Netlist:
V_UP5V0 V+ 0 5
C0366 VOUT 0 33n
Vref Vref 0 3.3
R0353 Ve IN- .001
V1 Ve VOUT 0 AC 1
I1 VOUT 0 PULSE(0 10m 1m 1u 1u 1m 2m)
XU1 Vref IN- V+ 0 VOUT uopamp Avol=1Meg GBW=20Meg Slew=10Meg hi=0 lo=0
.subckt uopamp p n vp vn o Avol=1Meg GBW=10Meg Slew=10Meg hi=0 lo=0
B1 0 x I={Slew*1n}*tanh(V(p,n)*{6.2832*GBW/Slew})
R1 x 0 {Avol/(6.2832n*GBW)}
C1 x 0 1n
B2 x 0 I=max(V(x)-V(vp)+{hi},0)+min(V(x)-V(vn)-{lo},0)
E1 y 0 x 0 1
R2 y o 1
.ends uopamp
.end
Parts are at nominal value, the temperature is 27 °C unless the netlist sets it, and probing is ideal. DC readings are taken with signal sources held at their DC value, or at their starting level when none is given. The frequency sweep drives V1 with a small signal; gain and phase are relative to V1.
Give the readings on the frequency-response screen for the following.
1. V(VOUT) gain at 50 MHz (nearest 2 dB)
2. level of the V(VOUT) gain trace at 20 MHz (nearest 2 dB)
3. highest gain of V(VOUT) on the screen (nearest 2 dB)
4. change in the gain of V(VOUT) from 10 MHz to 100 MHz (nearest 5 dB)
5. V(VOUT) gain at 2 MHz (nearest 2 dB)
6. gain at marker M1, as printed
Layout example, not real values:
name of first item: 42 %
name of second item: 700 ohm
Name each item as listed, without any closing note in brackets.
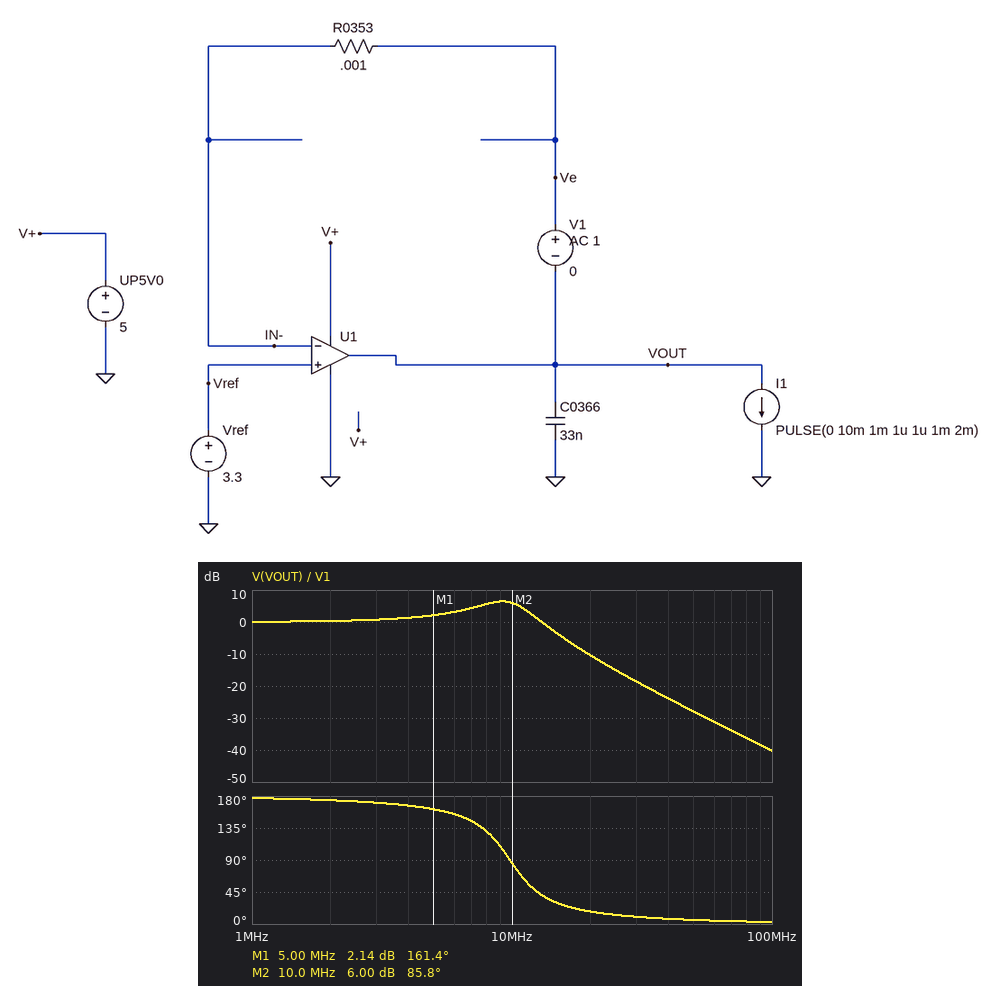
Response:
V(VOUT) gain at 50 MHz: -28 dB
level of the V(VOUT) gain trace at 20 MHz: -10 dB
highest gain of V(VOUT) on the screen: 6 dB
change in the gain of V(VOUT) from 10 MHz to 100 MHz: -45 dB
V(VOUT) gain at 2 MHz: 0 dB
gain at marker M1, as printed: 2.14 dB
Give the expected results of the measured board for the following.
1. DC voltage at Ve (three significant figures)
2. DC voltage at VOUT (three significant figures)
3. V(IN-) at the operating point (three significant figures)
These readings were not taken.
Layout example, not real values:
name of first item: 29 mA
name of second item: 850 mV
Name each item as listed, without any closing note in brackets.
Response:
DC voltage at Ve: 3.30 V
DC voltage at VOUT: 3.30 V
V(IN-) at the operating point: 3.30 V
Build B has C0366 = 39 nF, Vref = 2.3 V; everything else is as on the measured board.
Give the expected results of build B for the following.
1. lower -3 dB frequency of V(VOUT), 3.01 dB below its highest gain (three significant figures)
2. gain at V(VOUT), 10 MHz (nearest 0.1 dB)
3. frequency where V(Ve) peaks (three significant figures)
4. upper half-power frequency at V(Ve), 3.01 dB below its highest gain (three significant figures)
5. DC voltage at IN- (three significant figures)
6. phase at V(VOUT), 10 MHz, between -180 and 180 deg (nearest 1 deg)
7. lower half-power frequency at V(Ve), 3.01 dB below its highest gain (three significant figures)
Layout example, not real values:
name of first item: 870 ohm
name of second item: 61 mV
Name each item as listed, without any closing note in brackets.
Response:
lower -3 dB frequency of V(VOUT), 3.01 dB below its highest gain: 6.11 MHz
gain at V(VOUT), 10 MHz: 5.2 dB
frequency where V(Ve) peaks: 9.45 MHz
upper half-power frequency at V(Ve), 3.01 dB below its highest gain: 12.9 MHz
DC voltage at IN-: 2.30 V
phase at V(VOUT), 10 MHz, between -180 and 180 deg: 66 deg
lower half-power frequency at V(Ve), 3.01 dB below its highest gain: 7.71 MHz
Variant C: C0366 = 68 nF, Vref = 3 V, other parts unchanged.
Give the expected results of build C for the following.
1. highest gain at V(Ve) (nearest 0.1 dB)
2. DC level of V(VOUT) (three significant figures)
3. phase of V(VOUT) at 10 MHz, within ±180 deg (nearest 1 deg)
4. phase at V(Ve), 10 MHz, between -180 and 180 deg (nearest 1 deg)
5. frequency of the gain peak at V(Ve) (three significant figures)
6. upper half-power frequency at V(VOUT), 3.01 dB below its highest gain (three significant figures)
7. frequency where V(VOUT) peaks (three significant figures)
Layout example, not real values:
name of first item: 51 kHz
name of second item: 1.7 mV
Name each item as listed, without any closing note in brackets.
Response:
highest gain at V(Ve): 9.9 dB
DC level of V(VOUT): 3.00 V
phase of V(VOUT) at 10 MHz, within ±180 deg: 24 deg
phase at V(Ve), 10 MHz, between -180 and 180 deg: 11 deg
frequency of the gain peak at V(Ve): 7.03 MHz
upper half-power frequency at V(VOUT), 3.01 dB below its highest gain: 7.74 MHz
frequency where V(VOUT) peaks: 6.64 MHz
